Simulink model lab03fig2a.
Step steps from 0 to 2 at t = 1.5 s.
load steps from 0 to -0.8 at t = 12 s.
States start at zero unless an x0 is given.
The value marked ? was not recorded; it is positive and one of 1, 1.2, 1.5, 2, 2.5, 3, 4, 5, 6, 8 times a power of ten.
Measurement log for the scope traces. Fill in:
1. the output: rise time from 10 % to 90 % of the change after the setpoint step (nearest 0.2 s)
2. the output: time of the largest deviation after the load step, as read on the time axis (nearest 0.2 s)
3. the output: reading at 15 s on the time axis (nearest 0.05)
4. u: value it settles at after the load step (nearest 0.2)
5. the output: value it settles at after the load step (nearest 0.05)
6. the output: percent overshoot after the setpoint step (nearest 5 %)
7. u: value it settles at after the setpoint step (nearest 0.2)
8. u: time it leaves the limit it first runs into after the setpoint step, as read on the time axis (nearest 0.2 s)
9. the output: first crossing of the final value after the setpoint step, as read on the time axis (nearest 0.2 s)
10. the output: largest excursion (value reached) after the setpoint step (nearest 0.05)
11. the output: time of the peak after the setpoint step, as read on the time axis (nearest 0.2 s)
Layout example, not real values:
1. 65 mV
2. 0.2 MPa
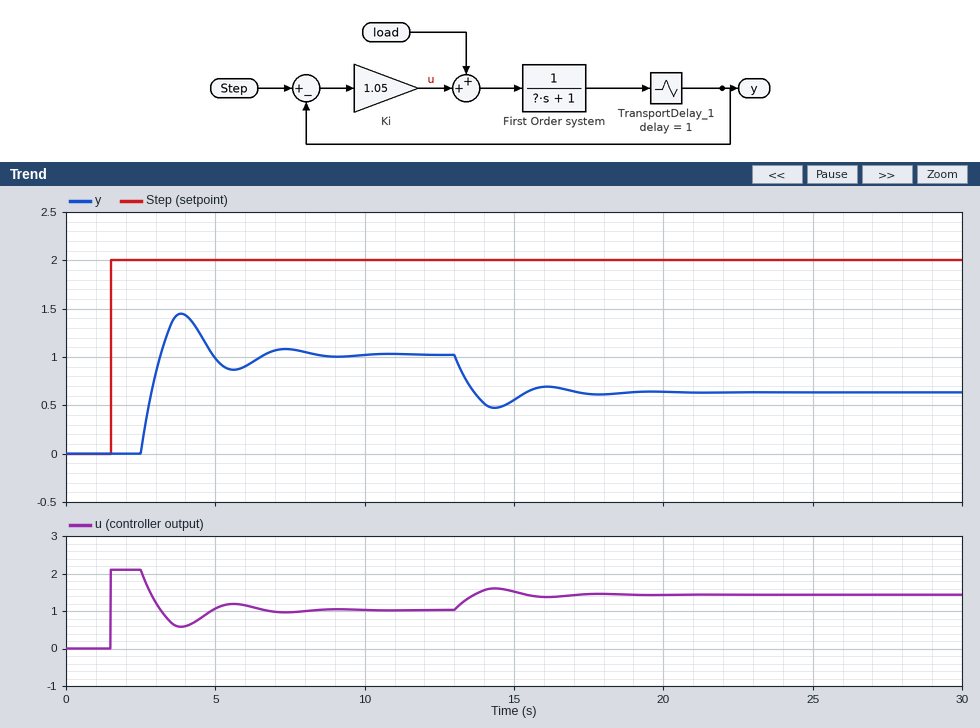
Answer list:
1. 0.6 s
2. 14.4 s
3. 0.55
4. 1.4
5. 0.65
6. 40 %
7. 1.0
8. 2.6 s
9. 3.2 s
10. 1.45
11. 3.8 s
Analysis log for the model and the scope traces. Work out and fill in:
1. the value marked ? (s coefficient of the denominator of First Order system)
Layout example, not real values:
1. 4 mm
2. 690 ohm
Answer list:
1. 1
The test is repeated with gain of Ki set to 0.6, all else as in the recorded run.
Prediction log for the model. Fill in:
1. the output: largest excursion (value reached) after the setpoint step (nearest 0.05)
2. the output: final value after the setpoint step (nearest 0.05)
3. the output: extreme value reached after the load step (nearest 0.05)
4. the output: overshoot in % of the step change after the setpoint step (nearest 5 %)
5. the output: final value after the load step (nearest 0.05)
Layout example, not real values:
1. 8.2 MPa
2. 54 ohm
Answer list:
1. 0.85
2. 0.75
3. 0.15
4. 15 %
5. 0.25
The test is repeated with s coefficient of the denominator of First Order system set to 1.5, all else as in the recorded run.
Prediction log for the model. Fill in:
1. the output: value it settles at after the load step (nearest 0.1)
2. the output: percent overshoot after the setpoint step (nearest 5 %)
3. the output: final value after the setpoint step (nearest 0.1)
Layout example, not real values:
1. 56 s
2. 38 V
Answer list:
1. 0.6
2. 20 %
3. 1.0
